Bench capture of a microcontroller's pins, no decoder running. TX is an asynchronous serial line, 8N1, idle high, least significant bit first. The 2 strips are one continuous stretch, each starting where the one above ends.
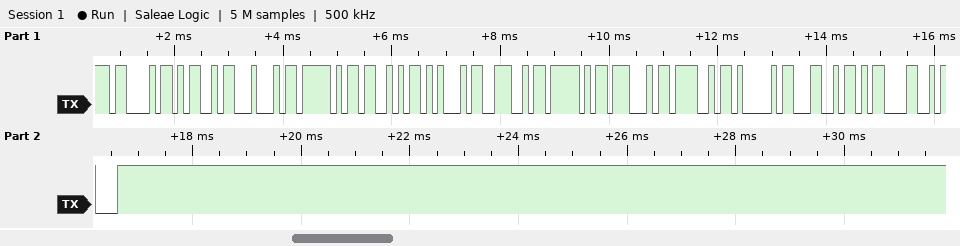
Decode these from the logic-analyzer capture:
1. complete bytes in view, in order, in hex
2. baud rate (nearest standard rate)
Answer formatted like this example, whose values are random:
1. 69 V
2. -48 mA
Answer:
1. 0x43 0x4D 0x44 0x5F 0x53 0x45 0x4E 0x5F 0x47 0x4F 0x41 0x4C 0x0D 0x0A
2. 9600 baud
